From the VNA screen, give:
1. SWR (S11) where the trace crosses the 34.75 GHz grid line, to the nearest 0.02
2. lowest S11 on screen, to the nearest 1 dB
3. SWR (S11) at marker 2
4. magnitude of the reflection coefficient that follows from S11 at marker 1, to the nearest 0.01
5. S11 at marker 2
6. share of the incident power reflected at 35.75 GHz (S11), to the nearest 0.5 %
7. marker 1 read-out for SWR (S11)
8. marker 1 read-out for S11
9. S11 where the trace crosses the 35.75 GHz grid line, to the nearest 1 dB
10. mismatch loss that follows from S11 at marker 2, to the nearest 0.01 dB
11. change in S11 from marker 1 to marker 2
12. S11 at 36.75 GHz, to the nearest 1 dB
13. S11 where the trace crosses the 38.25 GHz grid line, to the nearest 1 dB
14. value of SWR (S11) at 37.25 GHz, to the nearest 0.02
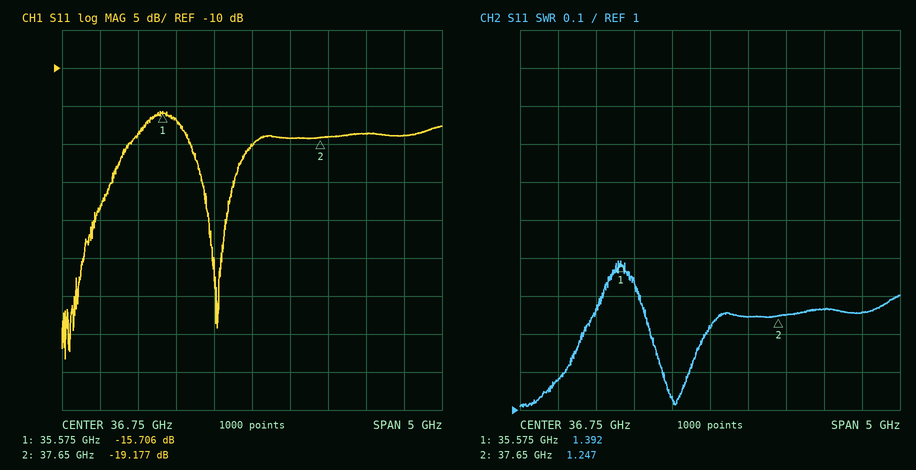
1.08
-48 dB
1.247
0.16
-19.177 dB
2.0 %
1.392
-15.706 dB
-17 dB
0.05 dB
-3.471 dB
-20 dB
-19 dB
1.24
